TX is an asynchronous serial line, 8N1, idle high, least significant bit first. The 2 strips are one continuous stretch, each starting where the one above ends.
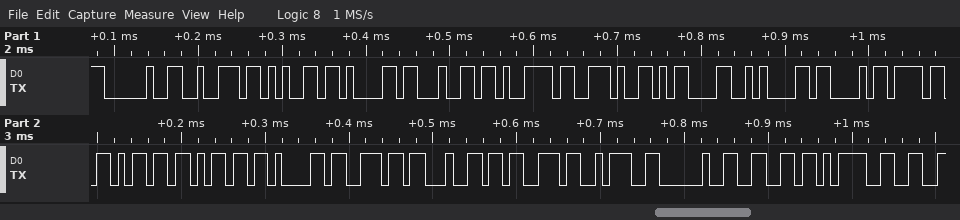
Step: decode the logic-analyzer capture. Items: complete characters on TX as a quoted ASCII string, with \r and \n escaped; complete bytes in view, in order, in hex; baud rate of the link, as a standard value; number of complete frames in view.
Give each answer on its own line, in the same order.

" ready.\r\nCommands: f="
20 72 65 61 64 79 2E 0D 0A 43 6F 6D 6D 61 6E 64 73 3A 20 66 3D
115200 baud
21
